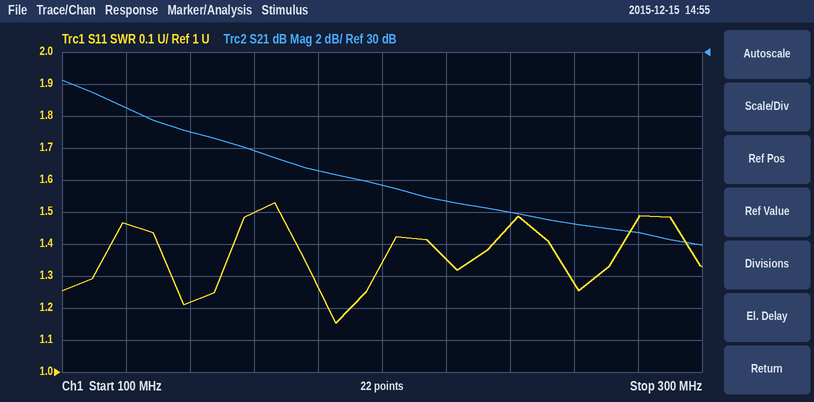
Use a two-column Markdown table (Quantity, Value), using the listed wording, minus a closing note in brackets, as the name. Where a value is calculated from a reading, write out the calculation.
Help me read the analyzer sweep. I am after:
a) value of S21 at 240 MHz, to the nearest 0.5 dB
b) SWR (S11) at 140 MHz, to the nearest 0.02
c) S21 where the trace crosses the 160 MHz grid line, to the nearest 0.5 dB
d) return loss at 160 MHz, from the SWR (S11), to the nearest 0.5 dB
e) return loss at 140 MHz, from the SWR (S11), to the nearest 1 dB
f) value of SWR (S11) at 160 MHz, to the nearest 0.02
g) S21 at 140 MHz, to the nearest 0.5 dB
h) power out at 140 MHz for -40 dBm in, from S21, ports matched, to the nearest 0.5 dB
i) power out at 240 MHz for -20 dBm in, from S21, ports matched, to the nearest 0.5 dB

| Quantity | Value |
|---|---|
| value of S21 at 240 MHz, to the nearest 0.5 dB | 20.0 dB |
| SWR (S11) at 140 MHz, to the nearest 0.02 | 1.22 |
| S21 where the trace crosses the 160 MHz grid line, to the nearest 0.5 dB | 24.0 dB |
| return loss at 160 MHz, from the SWR (S11), to the nearest 0.5 dB | −20 log10((1.5 − 1)/(1.5 + 1)) ≈ 14.0 dB |
| return loss at 140 MHz, from the SWR (S11), to the nearest 1 dB | −20 log10((1.22 − 1)/(1.22 + 1)) ≈ 20 dB |
| value of SWR (S11) at 160 MHz, to the nearest 0.02 | 1.50 |
| S21 at 140 MHz, to the nearest 0.5 dB | 25.0 dB |
| power out at 140 MHz for -40 dBm in, from S21, ports matched, to the nearest 0.5 dB | -40 dBm + (25.0 dB) = -15.0 dBm |
| power out at 240 MHz for -20 dBm in, from S21, ports matched, to the nearest 0.5 dB | -20 dBm + (20.0 dB) = 0.0 dBm |
